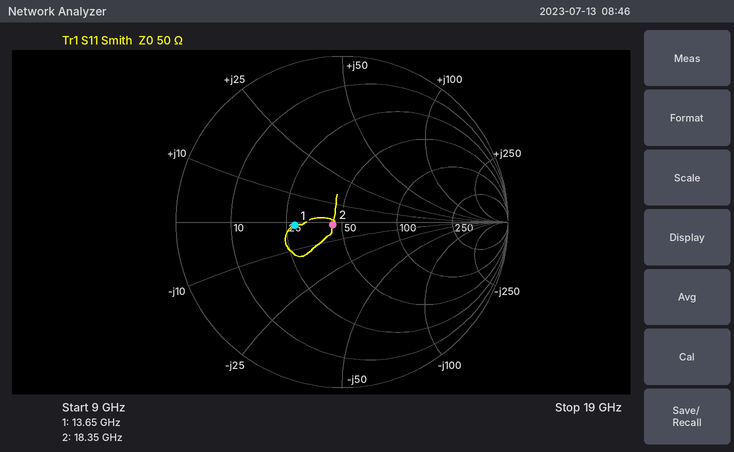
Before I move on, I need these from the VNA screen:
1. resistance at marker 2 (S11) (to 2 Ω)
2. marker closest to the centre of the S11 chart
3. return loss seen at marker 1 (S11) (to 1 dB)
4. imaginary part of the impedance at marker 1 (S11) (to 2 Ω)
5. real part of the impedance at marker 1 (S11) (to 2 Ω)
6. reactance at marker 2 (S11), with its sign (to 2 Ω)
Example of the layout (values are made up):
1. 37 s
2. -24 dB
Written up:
1. 44 Ω
2. marker 2
3. 11 dB
4. -2 Ω
5. 28 Ω
6. -2 Ω
